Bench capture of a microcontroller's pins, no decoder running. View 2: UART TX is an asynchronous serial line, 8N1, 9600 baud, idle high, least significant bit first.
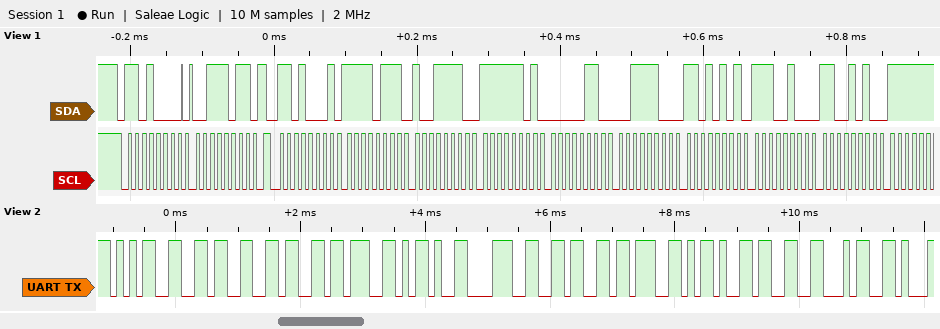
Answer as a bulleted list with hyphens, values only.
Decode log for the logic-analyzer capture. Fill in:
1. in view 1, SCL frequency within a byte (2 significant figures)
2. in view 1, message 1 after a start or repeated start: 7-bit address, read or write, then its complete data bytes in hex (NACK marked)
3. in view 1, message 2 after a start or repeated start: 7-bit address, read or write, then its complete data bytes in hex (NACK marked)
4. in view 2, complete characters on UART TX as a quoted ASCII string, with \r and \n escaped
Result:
- 100 kHz
- 0x68 write: 3B
- 0x68 read: F7 9E FD 06 3C D5 E4 CA
- "566;-86;-34"
